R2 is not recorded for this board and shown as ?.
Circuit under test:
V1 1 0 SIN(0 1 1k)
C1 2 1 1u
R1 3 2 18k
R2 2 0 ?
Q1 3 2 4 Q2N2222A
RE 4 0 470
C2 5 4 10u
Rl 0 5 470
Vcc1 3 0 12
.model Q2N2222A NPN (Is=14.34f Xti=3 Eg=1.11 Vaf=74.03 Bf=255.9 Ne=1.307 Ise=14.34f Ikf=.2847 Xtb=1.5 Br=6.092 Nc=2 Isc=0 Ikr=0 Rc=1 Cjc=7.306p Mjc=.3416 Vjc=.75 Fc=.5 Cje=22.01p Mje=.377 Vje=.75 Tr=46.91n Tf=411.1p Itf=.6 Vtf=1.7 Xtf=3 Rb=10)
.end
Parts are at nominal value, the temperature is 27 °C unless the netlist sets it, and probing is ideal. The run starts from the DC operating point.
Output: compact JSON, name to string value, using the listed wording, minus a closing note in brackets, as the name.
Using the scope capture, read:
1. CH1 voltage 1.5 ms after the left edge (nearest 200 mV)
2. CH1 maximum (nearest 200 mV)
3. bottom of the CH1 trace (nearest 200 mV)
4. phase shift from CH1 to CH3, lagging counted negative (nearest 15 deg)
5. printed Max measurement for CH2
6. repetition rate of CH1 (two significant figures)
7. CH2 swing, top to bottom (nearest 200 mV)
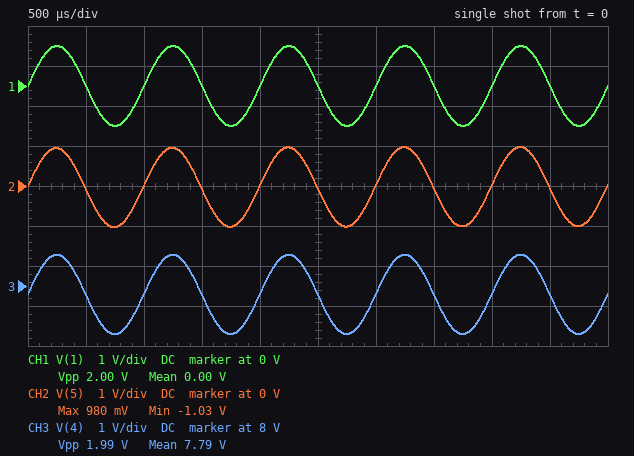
{"CH1 voltage 1.5 ms after the left edge": "0 V", "CH1 maximum": "1.0 V", "bottom of the CH1 trace": "-1.0 V", "phase shift from CH1 to CH3, lagging counted negative": "0 deg", "printed Max measurement for CH2": "980 mV", "repetition rate of CH1": "1.0 kHz", "CH2 swing, top to bottom": "2.0 V"}
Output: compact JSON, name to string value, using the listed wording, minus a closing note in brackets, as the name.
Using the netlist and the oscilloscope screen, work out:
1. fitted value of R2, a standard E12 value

{"fitted value of R2, a standard E12 value": "82 kΩ"}
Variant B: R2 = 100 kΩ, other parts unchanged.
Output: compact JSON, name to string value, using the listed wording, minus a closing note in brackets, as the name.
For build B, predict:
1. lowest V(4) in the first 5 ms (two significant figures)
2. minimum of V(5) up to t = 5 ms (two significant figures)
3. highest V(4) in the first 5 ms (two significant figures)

{"lowest V(4) in the first 5 ms": "7.0 V", "minimum of V(5) up to t = 5 ms": "-1.0 V", "highest V(4) in the first 5 ms": "9.0 V"}
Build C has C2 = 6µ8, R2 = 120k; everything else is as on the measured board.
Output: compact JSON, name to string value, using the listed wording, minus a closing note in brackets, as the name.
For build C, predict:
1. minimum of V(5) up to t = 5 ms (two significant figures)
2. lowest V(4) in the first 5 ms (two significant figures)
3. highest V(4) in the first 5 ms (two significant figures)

{"minimum of V(5) up to t = 5 ms": "-1.0 V", "lowest V(4) in the first 5 ms": "7.2 V", "highest V(4) in the first 5 ms": "9.2 V"}
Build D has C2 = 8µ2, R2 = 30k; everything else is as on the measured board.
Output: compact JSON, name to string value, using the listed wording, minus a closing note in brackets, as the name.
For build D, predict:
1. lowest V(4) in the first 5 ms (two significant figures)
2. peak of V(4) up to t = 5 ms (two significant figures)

{"lowest V(4) in the first 5 ms": "5.0 V", "peak of V(4) up to t = 5 ms": "7.0 V"}
